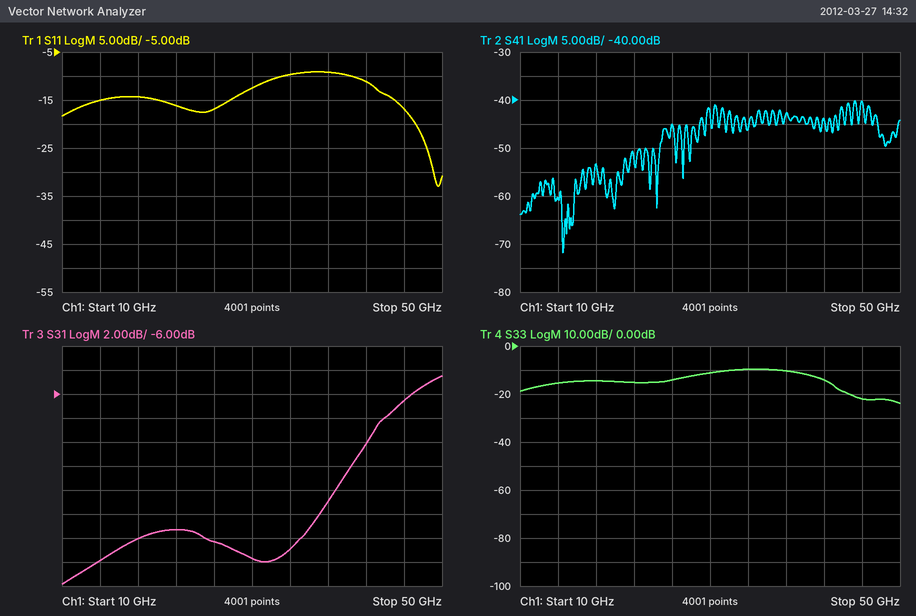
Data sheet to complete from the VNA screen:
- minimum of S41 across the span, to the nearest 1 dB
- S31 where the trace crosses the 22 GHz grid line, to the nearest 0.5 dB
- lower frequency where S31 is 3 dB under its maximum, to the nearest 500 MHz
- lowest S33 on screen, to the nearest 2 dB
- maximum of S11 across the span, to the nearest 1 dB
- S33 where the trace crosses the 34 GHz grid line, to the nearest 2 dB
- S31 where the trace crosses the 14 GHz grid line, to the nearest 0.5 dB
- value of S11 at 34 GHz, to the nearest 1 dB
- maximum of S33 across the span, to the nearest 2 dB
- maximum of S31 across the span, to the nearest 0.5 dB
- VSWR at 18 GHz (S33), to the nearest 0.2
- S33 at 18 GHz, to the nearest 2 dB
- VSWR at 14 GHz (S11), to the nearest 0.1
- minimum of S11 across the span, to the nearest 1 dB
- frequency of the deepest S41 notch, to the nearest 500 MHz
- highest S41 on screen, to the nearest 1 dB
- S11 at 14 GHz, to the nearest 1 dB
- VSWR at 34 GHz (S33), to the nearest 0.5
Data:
-72 dB
-17.5 dB
44.5 GHz
-24 dB
-9 dB
-10 dB
-20.0 dB
-10 dB
-10 dB
-4.5 dB
1.4
-14 dB
1.4
-33 dB
14.5 GHz
-40 dB
-15 dB
2.0
